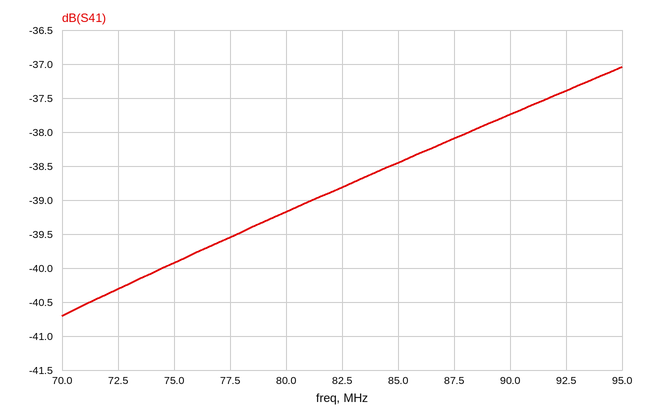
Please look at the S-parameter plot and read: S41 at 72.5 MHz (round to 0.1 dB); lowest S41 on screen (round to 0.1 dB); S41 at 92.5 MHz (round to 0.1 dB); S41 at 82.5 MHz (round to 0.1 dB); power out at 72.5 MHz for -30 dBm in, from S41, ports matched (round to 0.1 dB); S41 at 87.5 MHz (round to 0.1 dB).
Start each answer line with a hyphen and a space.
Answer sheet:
- -40.3 dB
- -40.7 dB
- -37.4 dB
- -38.8 dB
- -70.3 dBm
- -38.1 dB
